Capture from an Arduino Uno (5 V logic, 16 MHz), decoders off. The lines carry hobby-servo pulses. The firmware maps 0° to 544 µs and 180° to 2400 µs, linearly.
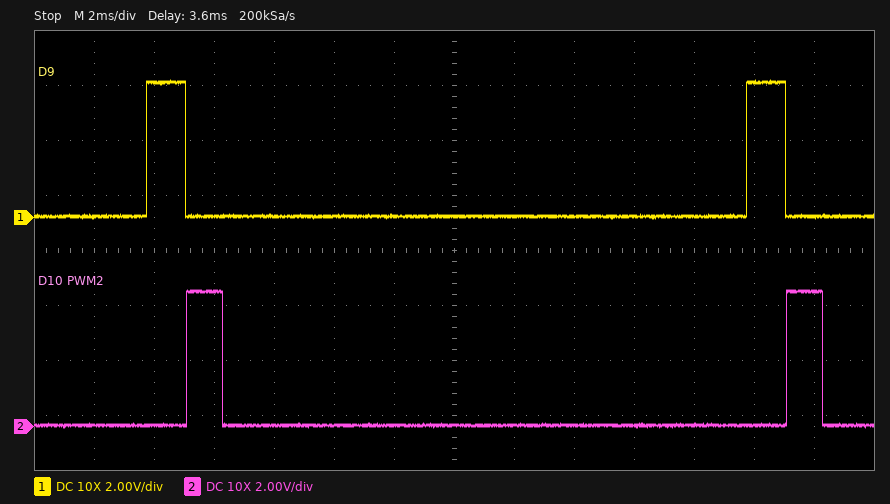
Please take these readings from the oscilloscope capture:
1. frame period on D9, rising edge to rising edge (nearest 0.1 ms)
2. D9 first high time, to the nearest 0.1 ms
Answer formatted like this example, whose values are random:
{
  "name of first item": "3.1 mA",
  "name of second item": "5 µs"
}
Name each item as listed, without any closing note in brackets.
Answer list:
{
  "frame period on D9, rising edge to rising edge": "20.0 ms",
  "D9 first high time, to the nearest 0.1 ms": "1.3 ms"
}
